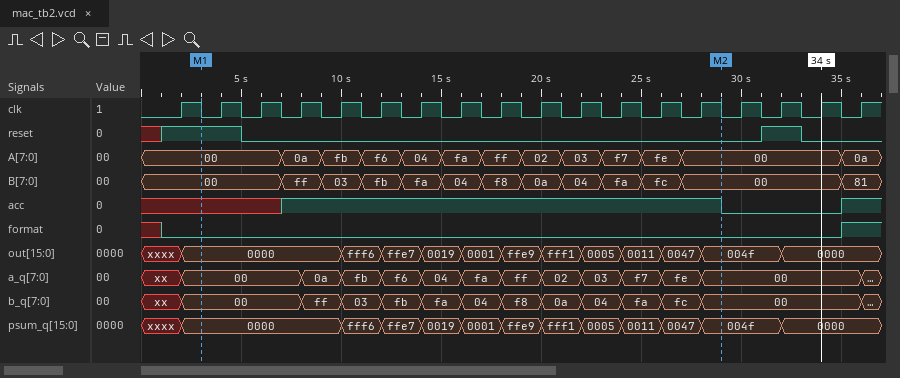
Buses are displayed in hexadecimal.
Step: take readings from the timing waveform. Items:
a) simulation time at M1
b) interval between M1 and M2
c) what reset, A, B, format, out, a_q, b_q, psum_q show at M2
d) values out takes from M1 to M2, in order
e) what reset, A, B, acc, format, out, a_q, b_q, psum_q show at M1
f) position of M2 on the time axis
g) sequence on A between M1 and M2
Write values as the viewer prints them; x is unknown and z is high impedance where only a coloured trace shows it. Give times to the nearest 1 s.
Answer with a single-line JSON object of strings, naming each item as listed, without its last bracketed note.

{"simulation time at M1": "3 s", "interval between M1 and M2": "26 s", "what reset, A, B, format, out, a_q, b_q, psum_q show at M2": "reset=0, A=00, B=00, format=0, out=004f, a_q=00, b_q=00, psum_q=004f", "values out takes from M1 to M2, in order": "0000, fff6, ffe7, 0019, 0001, ffe9, fff1, 0005, 0011, 0047, 004f", "what reset, A, B, acc, format, out, a_q, b_q, psum_q show at M1": "reset=1, A=00, B=00, acc=x, format=0, out=0000, a_q=00, b_q=00, psum_q=0000", "position of M2 on the time axis": "29 s", "sequence on A between M1 and M2": "00, 0a, fb, f6, 04, fa, ff, 02, 03, f7, fe, 00"}
